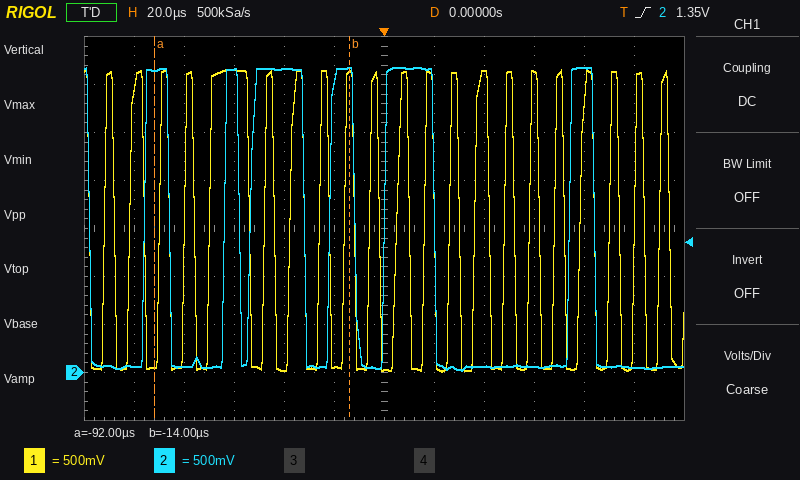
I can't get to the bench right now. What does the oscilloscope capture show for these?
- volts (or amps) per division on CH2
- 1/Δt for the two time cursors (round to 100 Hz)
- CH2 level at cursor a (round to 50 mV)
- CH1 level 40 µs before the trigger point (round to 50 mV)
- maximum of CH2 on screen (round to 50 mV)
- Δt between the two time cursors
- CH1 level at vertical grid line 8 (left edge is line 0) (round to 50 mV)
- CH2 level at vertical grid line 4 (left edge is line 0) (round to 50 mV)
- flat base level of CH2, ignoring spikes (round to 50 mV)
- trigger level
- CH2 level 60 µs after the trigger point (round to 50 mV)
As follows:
500 mV
12.8 kHz
3.15 V
50 mV
3.20 V
78 µs
3.10 V
3.15 V
50 mV
1.35 V
50 mV
